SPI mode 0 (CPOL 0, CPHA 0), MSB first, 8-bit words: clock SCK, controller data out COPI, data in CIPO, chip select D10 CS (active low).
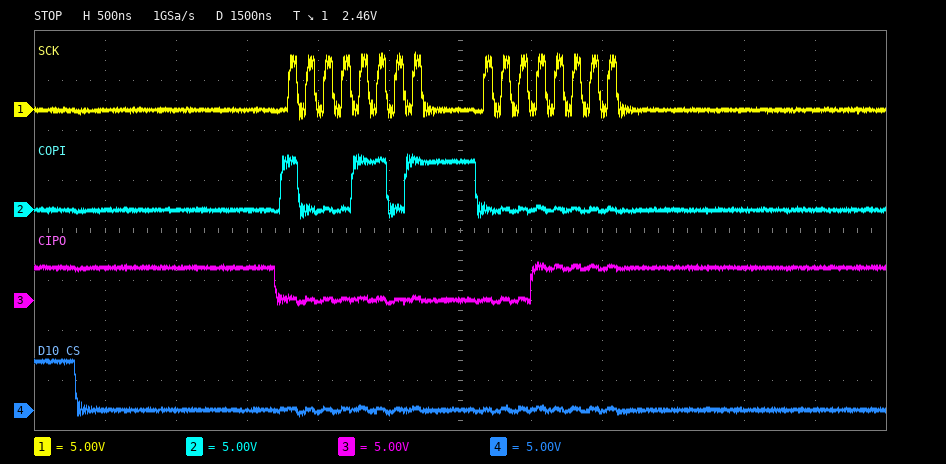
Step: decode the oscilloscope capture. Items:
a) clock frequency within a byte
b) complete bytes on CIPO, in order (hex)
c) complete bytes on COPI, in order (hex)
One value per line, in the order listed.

8 MHz
00 1F
8D 00
